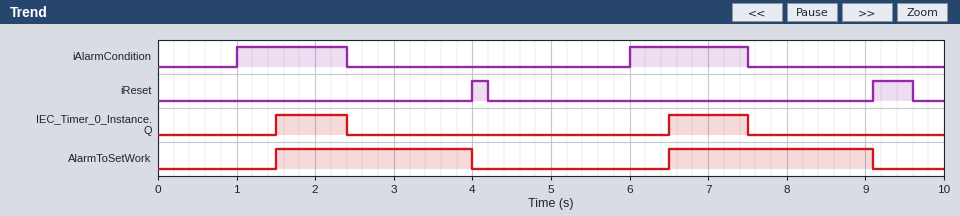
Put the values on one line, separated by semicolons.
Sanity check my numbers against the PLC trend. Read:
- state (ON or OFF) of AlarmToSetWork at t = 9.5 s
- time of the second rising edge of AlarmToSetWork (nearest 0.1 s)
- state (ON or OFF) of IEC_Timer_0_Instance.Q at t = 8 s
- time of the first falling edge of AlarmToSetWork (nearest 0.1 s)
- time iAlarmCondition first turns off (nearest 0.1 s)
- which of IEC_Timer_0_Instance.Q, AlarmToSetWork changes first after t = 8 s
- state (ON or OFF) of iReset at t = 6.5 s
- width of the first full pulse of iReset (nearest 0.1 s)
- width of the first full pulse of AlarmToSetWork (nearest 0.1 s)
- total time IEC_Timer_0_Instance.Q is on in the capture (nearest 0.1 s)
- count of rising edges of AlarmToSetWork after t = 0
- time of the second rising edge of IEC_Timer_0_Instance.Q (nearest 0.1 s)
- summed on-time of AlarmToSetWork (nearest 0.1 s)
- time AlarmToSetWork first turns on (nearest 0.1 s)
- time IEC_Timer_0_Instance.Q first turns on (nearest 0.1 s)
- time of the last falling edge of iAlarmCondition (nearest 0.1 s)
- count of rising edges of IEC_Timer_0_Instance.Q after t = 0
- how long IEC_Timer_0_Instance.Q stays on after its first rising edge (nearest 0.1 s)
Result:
OFF; 6.5 s; OFF; 4.0 s; 2.4 s; AlarmToSetWork; OFF; 0.2 s; 2.5 s; 1.9 s; 2; 6.5 s; 5.1 s; 1.5 s; 1.5 s; 7.5 s; 2; 0.9 s
